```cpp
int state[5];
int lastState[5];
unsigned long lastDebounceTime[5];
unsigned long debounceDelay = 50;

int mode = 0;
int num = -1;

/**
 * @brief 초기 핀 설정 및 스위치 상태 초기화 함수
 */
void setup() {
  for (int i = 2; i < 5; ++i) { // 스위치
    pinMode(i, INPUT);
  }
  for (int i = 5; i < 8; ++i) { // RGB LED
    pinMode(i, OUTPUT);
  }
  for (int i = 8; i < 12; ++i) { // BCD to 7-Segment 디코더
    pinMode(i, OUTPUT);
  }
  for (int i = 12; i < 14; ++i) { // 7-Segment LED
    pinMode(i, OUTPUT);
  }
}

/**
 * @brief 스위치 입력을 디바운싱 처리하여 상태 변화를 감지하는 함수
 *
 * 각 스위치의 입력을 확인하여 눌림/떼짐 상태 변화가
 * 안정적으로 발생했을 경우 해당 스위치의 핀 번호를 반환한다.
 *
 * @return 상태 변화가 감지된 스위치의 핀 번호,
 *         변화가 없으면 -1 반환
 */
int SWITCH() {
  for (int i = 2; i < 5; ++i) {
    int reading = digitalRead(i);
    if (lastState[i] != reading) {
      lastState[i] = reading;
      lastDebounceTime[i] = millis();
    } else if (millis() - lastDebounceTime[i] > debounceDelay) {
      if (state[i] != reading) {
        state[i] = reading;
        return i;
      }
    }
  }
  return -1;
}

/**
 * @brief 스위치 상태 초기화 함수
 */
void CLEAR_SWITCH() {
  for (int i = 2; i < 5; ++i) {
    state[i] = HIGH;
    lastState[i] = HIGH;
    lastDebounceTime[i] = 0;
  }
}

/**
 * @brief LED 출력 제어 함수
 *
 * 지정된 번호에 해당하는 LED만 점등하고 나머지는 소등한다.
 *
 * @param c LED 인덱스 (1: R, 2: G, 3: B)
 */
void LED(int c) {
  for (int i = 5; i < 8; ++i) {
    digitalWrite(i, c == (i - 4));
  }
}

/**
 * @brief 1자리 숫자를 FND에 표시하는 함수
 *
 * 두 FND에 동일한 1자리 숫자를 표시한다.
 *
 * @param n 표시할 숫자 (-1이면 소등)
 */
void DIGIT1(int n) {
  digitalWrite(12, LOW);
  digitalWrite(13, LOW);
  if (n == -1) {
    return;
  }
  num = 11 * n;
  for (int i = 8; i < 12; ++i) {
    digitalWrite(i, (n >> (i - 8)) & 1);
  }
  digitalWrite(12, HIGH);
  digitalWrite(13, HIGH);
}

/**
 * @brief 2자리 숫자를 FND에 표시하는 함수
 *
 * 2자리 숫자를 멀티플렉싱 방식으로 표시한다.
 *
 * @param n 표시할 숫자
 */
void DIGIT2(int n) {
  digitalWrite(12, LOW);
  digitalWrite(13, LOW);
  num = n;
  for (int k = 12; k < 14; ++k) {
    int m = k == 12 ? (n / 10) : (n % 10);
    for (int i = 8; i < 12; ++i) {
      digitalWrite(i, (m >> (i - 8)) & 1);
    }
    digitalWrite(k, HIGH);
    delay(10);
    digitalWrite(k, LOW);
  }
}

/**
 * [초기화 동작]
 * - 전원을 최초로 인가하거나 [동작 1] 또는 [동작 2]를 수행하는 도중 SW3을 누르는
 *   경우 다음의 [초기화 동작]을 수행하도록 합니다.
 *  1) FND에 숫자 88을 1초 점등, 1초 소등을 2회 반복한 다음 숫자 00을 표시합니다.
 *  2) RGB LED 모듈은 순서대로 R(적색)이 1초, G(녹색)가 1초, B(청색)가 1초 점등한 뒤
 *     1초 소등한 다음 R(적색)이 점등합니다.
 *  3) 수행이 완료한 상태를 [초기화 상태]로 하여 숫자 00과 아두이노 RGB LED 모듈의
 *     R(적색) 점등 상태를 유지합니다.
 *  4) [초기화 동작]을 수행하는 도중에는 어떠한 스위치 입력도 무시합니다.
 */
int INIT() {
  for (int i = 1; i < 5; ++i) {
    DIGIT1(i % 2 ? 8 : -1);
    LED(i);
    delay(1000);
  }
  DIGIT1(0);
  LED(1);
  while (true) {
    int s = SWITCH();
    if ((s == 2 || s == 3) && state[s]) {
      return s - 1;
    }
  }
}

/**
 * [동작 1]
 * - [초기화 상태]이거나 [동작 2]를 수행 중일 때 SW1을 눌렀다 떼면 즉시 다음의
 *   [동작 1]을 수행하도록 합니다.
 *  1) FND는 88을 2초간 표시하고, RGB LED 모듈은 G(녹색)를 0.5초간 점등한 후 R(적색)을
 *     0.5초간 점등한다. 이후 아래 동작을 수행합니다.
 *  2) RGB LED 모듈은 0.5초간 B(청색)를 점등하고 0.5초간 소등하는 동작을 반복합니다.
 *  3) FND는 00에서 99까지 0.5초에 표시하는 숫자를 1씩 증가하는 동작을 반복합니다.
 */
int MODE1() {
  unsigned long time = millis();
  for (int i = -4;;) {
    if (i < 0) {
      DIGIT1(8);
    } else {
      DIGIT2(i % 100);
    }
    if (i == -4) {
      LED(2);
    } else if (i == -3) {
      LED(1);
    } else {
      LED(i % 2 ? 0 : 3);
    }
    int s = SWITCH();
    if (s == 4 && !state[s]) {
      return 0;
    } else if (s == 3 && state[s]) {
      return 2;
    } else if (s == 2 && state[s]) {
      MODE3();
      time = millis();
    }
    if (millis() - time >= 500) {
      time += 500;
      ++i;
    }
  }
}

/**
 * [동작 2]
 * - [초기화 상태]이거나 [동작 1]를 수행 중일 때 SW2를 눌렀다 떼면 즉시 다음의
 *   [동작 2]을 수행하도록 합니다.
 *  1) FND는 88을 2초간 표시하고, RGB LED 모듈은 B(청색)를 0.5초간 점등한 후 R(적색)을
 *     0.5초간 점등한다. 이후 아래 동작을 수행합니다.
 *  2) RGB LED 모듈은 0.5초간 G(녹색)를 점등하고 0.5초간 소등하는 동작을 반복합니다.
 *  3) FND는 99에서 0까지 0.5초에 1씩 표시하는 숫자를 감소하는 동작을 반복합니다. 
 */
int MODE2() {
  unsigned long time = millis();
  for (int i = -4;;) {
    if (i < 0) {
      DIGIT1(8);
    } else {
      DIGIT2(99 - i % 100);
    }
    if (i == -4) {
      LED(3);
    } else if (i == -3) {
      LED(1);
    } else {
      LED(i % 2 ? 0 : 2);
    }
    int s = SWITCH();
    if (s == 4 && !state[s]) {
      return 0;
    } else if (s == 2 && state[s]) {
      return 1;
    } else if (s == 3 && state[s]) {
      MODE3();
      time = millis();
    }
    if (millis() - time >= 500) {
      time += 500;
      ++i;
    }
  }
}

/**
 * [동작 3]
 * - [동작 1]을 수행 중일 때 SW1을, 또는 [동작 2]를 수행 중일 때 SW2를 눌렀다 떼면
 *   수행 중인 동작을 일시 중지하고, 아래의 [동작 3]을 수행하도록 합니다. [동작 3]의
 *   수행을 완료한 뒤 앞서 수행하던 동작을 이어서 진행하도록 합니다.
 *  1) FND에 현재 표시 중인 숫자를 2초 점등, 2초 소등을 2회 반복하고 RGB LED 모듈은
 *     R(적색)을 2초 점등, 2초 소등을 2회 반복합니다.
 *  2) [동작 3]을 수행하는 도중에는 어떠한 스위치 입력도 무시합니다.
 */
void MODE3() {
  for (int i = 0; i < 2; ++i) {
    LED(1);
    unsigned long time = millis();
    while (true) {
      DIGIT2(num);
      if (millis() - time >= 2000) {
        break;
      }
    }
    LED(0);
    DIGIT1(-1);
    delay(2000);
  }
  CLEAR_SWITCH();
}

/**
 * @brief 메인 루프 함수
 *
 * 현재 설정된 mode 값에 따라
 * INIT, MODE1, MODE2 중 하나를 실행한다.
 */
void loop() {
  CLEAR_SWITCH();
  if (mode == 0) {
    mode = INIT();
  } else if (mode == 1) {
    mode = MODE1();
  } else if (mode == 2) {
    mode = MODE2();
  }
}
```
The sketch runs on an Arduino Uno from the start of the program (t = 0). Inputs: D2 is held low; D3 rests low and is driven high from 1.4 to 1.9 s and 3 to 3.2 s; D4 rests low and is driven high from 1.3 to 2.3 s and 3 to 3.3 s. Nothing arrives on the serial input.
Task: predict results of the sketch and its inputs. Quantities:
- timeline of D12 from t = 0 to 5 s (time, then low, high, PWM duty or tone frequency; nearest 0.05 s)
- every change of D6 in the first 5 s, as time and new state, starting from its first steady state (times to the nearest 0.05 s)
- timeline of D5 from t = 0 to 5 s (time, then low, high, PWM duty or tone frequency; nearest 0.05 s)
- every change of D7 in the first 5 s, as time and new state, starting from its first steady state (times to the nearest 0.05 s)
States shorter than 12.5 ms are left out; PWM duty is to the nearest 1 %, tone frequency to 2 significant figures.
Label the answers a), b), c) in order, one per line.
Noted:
a) 0 s high; 1 s low; 2 s high; 3 s low; 4 s high
b) 0 s low; 1 s high; 2 s low
c) 0 s high; 1 s low; 4 s high
d) 0 s low; 2 s high; 3 s low
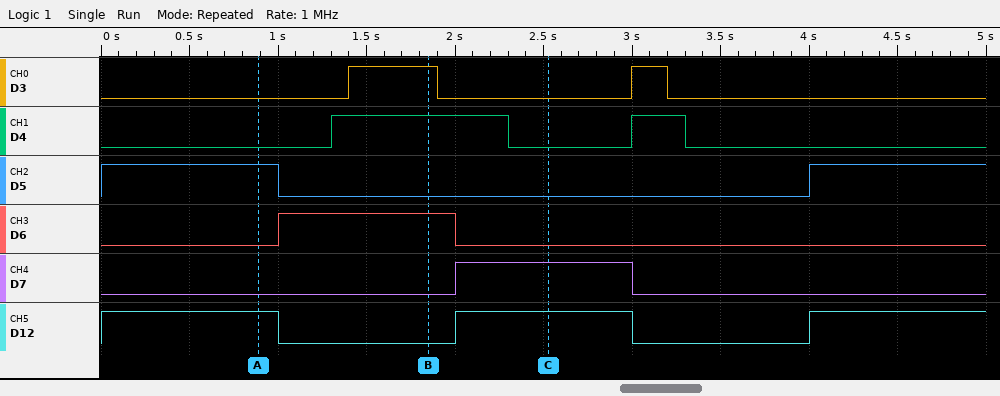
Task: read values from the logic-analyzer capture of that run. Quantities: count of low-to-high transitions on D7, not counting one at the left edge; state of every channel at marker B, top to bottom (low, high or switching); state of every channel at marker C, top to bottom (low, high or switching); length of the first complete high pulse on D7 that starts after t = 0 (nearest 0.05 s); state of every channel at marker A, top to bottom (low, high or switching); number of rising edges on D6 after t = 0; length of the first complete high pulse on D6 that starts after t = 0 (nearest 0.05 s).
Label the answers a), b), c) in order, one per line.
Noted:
a) 1
b) D3 high, D4 high, D5 low, D6 high, D7 low, D12 low
c) D3 low, D4 low, D5 low, D6 low, D7 high, D12 high
d) 1.00 s
e) D3 low, D4 low, D5 high, D6 low, D7 low, D12 high
f) 1
g) 1.00 s
